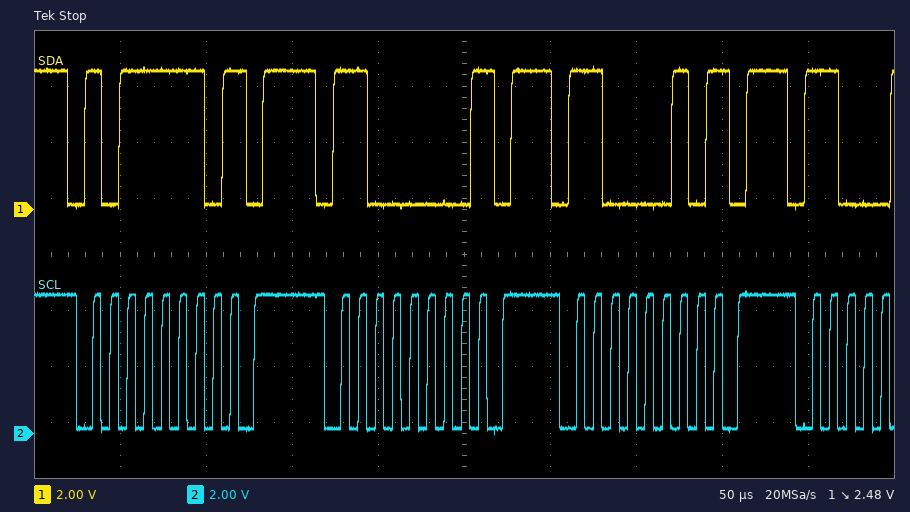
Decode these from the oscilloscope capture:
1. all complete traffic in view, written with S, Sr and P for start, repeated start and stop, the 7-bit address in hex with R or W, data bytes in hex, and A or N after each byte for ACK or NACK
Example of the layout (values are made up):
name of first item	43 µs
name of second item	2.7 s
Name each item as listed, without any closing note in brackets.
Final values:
all complete traffic in view, written with S, Sr and P for start, repeated start and stop, the 7-bit address in hex with R or W, data bytes in hex, and A or N after each byte for ACK or NACK	S 5FW N P S 60W N P S 61W N P
